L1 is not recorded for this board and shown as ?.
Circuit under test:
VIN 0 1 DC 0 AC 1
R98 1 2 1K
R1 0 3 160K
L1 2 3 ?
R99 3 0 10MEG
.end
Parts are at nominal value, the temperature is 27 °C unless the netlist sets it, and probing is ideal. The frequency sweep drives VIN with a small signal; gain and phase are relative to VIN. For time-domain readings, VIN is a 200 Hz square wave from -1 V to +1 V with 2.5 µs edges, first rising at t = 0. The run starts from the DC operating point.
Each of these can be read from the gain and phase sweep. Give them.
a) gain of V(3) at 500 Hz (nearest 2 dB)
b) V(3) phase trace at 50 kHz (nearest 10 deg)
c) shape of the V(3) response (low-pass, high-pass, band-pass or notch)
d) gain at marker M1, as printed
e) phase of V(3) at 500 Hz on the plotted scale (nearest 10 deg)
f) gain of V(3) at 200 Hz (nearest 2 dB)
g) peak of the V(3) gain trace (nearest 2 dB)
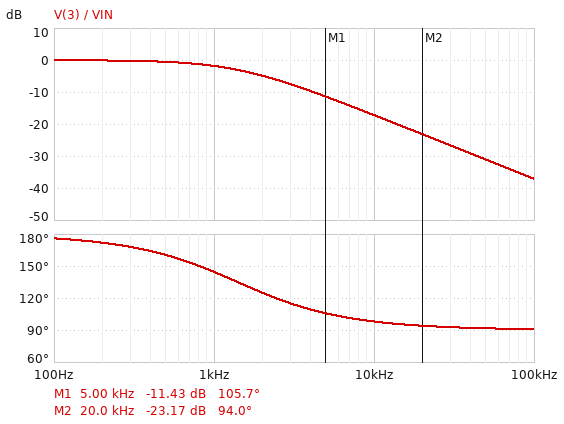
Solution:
0 dB
90 deg
low-pass
-11.43 dB
160 deg
0 dB
0 dB
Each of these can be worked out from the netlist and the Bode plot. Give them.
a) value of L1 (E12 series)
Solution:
18 H
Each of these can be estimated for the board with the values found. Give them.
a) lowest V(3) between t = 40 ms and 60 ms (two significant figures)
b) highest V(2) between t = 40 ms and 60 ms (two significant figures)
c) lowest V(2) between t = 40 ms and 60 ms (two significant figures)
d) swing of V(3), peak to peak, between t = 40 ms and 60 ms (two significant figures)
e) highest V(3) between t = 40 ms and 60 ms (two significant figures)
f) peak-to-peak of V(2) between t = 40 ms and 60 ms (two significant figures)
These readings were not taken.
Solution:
-990 mV
1.0 V
-1.0 V
2.0 V
990 mV
2.0 V
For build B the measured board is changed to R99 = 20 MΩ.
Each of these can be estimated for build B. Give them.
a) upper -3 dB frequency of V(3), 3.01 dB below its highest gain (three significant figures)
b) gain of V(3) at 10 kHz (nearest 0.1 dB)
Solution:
1.41 kHz
-17.1 dB
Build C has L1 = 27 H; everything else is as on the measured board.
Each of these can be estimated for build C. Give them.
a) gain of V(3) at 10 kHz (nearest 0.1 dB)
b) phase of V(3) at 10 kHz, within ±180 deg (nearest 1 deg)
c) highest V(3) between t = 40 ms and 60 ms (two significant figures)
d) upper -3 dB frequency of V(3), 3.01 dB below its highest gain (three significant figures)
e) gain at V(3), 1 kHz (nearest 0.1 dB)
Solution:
-20.7 dB
95 deg
990 mV
934 Hz
-3.4 dB
